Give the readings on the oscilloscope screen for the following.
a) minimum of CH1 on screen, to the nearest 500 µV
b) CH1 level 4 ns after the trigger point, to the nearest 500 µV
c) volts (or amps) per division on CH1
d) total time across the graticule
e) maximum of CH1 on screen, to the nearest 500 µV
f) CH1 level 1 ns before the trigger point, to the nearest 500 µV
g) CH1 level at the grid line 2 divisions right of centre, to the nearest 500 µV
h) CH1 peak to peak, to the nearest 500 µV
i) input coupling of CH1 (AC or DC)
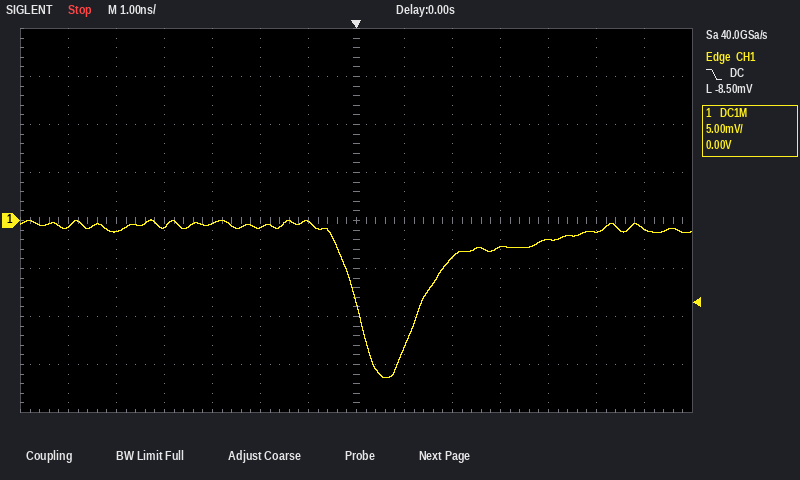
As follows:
-16.5 mV
-2.0 mV
5 mV
14 ns
0.0 mV
0.0 mV
-4.0 mV
16.5 mV
DC
